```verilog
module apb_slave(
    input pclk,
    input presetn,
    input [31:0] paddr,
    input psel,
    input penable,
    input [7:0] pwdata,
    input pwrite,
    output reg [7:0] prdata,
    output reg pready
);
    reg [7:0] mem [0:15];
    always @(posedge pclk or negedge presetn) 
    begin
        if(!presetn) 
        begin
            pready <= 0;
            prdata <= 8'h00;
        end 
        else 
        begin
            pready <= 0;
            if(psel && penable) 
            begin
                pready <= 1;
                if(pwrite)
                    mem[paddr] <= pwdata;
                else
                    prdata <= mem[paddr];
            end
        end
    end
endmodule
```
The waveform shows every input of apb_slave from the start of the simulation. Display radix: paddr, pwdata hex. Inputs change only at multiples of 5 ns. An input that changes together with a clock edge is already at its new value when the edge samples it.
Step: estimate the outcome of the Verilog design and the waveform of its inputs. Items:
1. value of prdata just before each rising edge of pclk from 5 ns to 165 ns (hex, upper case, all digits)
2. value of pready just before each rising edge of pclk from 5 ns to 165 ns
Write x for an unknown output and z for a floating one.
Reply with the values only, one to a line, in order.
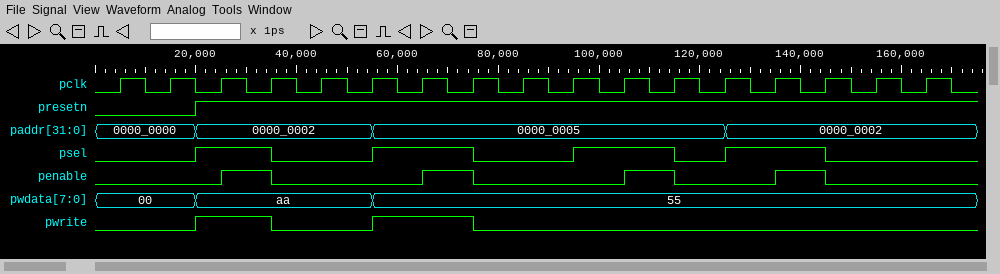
00, 00, 00, 00, 00, 00, 00, 00, 00, 00, 00, 55, 55, 55, AA, AA, AA
0 0 0 1 0 0 0 1 0 0 0 1 0 0 1 0 0
